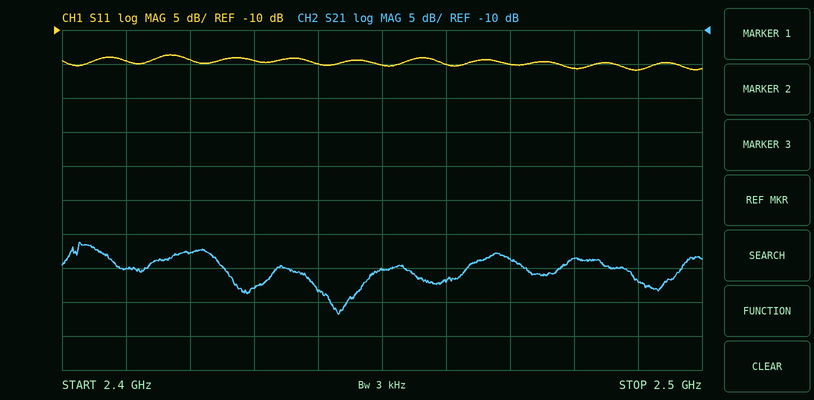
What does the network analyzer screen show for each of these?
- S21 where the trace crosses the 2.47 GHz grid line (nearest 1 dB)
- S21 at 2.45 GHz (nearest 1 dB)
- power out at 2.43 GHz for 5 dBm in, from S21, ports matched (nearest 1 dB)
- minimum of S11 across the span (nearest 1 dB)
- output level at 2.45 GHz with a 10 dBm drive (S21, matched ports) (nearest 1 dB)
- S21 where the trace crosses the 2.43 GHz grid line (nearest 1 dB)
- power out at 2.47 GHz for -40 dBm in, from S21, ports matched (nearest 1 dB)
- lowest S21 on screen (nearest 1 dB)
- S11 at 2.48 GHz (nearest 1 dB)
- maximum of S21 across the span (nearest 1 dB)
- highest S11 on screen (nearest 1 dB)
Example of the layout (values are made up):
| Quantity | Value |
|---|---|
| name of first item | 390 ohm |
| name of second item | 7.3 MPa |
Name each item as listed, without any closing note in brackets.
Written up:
| Quantity | Value |
|---|---|
| S21 where the trace crosses the 2.47 GHz grid line | -44 dB |
| S21 at 2.45 GHz | -45 dB |
| power out at 2.43 GHz for 5 dBm in, from S21, ports matched | -43 dBm |
| minimum of S11 across the span | -16 dB |
| output level at 2.45 GHz with a 10 dBm drive (S21, matched ports) | -35 dBm |
| S21 where the trace crosses the 2.43 GHz grid line | -48 dB |
| power out at 2.47 GHz for -40 dBm in, from S21, ports matched | -84 dBm |
| lowest S21 on screen | -52 dB |
| S11 at 2.48 GHz | -16 dB |
| maximum of S21 across the span | -41 dB |
| highest S11 on screen | -14 dB |
